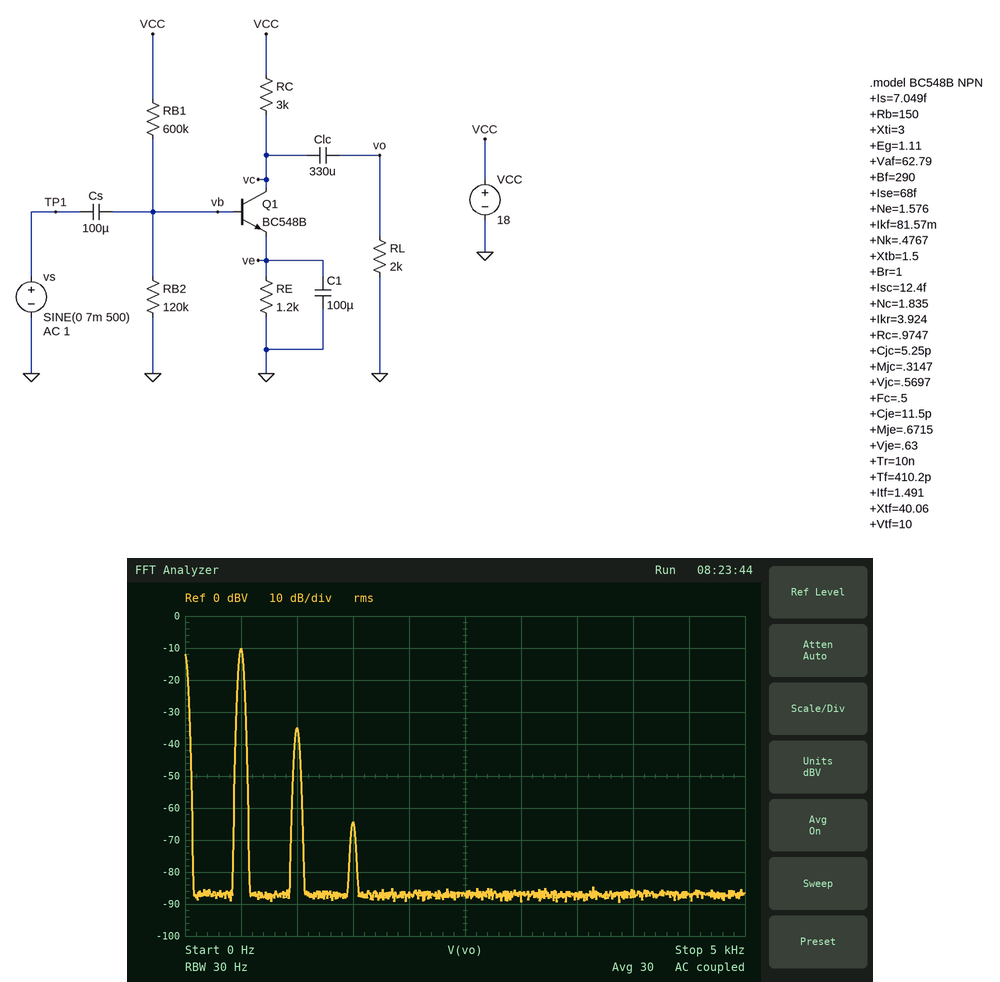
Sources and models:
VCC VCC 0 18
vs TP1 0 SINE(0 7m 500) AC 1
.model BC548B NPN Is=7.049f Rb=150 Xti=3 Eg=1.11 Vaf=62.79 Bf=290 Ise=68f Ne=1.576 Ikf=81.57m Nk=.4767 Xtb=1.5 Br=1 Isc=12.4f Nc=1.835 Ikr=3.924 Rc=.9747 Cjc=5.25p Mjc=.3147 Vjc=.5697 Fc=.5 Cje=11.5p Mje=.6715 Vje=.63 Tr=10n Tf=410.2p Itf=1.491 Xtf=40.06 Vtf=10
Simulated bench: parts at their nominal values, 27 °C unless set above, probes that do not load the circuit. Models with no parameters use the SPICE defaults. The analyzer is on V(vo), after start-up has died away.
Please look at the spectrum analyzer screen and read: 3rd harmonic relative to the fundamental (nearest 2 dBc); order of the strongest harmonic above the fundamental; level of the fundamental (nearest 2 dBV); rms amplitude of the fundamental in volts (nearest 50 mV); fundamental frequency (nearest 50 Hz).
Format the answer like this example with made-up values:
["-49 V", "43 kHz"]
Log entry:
["-54 dBc", "2", "-10 dBV", "300 mV", "500 Hz"]
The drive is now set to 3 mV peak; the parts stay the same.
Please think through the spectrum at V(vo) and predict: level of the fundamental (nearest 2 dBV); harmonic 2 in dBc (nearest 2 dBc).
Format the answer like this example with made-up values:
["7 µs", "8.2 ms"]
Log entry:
["-18 dBV", "-32 dBc"]
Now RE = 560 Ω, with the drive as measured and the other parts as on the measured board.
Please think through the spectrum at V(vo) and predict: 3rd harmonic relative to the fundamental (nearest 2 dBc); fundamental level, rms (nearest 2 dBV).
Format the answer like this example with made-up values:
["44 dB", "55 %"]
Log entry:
["-58 dBc", "-6 dBV"]
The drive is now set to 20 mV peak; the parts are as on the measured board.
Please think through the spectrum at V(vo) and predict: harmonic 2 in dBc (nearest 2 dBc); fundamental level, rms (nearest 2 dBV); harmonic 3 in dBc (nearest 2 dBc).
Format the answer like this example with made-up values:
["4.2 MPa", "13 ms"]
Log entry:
["-16 dBc", "-2 dBV", "-36 dBc"]
